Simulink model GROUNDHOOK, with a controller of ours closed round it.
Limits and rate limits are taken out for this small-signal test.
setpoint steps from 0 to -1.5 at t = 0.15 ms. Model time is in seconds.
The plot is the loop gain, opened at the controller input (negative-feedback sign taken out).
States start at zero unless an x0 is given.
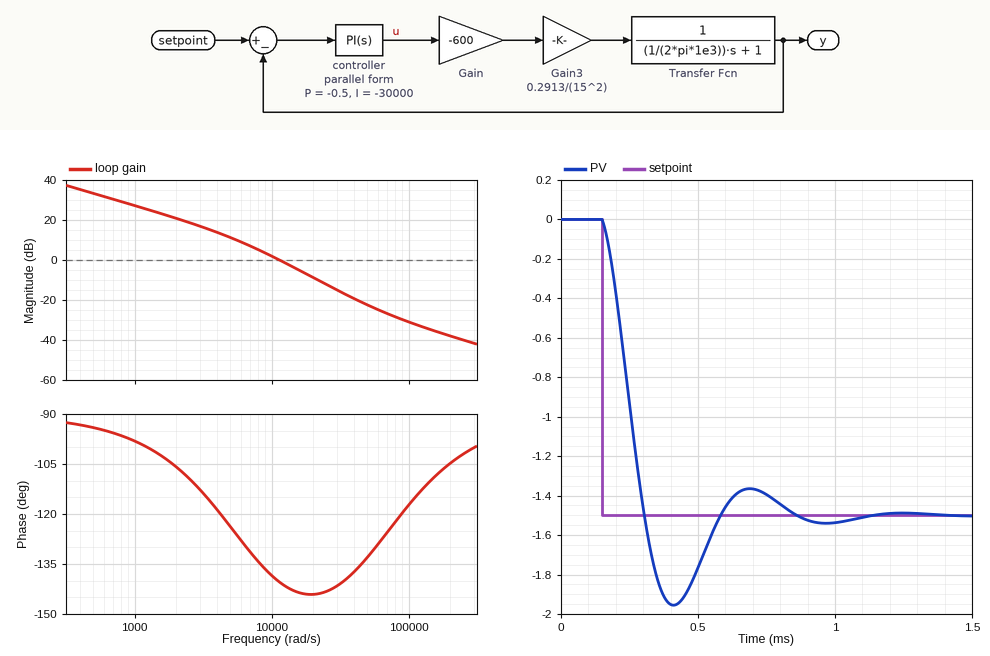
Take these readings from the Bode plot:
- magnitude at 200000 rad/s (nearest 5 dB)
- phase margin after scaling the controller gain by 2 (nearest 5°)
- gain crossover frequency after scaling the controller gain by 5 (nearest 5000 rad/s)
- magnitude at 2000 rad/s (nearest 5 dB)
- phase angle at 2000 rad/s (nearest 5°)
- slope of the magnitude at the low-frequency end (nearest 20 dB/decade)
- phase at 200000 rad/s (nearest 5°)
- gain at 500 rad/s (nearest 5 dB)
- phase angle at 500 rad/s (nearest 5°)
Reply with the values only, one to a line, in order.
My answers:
-40 dB
35°
30000 rad/s
20 dB
-105°
-20 dB/decade
-105°
35 dB
-95°
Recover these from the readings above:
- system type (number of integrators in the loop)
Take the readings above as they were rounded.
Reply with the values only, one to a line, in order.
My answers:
1
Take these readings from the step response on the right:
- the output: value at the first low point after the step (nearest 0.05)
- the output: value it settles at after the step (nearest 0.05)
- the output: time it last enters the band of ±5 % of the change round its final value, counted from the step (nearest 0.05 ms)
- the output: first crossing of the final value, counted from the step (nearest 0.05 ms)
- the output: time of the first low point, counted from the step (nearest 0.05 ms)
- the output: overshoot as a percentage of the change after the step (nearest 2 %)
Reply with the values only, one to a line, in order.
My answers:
-1.95
-1.50
0.65 ms
0.15 ms
0.25 ms
30 %
